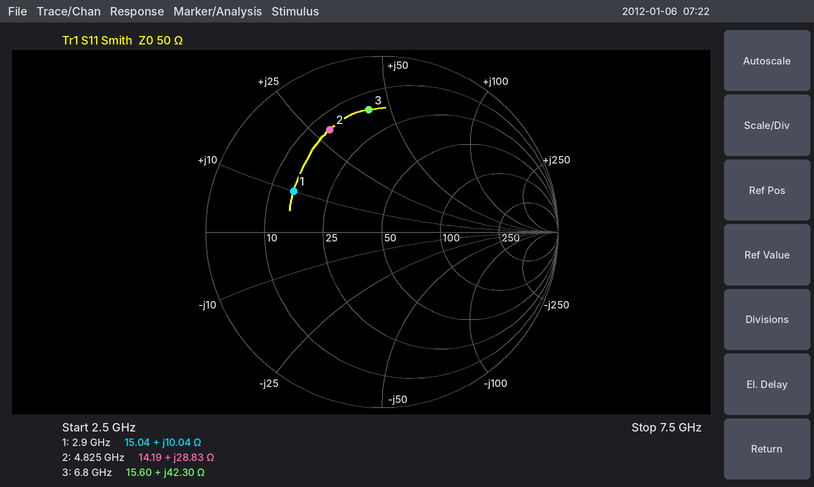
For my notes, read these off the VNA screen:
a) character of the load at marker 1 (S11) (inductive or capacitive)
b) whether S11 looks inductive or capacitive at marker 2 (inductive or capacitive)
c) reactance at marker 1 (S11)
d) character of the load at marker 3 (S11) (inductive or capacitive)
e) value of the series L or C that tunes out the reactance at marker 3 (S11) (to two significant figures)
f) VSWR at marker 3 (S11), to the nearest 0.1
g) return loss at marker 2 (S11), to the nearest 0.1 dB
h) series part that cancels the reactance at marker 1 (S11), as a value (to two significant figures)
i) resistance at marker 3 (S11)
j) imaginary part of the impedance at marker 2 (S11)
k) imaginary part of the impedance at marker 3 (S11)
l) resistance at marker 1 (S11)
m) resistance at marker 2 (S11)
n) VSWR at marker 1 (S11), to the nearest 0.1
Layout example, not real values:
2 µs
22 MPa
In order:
inductive
inductive
+10.04 Ω
inductive
550 fF
5.6
3.7 dB
5.5 pF
15.60 Ω
+28.83 Ω
+42.30 Ω
15.04 Ω
14.19 Ω
3.5
